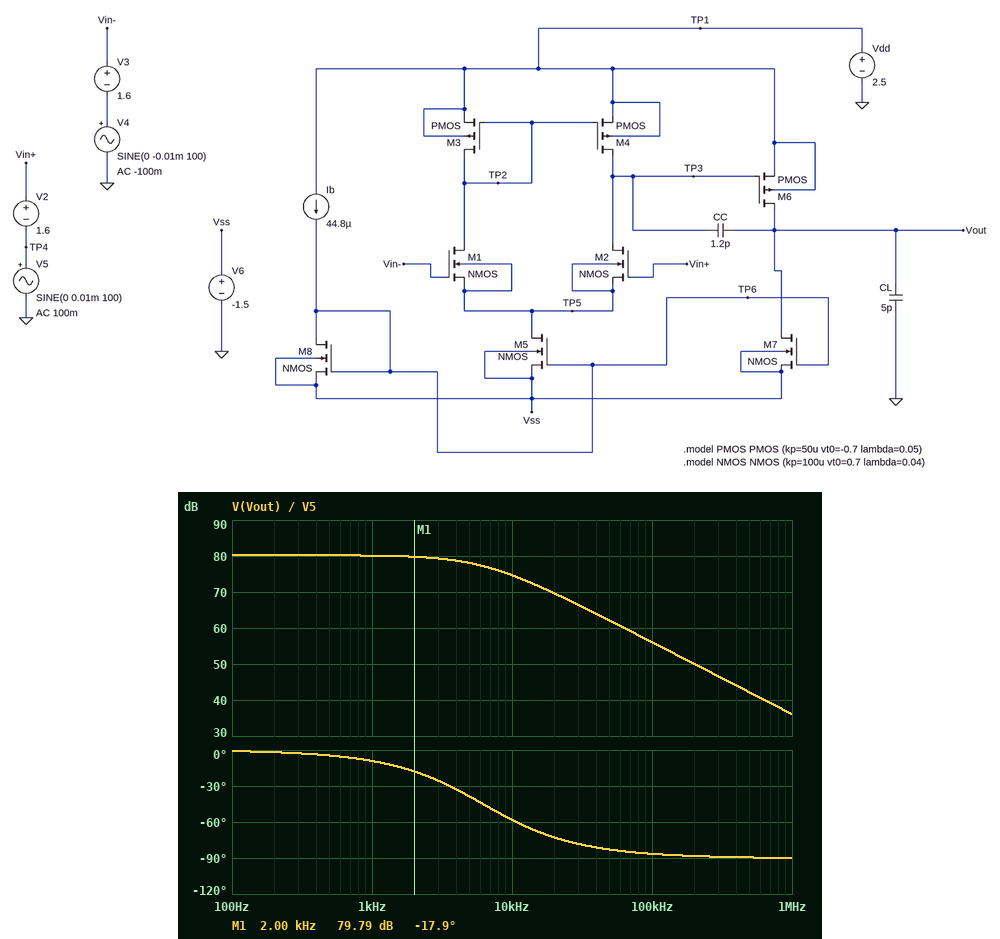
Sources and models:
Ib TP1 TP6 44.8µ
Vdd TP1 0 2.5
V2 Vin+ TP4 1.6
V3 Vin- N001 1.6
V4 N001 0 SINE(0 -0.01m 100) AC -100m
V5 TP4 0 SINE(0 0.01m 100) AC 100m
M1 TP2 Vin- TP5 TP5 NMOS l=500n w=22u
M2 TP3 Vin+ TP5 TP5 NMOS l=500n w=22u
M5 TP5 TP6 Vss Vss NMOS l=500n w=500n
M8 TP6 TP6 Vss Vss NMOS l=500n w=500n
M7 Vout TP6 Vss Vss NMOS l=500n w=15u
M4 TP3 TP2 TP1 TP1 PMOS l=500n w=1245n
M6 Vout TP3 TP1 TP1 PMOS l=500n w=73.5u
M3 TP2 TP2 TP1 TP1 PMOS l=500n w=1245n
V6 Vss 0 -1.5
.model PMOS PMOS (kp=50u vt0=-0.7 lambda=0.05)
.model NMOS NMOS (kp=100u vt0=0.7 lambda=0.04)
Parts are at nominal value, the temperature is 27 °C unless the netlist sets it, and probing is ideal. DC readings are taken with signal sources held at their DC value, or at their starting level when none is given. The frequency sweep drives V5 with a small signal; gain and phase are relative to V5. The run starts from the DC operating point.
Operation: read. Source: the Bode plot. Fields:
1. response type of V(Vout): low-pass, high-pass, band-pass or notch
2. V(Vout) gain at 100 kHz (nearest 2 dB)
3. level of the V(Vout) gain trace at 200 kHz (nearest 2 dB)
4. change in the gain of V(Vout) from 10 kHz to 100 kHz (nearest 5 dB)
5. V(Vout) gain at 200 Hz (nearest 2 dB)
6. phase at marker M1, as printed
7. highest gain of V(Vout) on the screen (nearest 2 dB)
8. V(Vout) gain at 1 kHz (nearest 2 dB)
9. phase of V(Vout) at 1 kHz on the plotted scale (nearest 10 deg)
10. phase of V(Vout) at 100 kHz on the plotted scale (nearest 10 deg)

low-pass
56 dB
50 dB
-20 dB
80 dB
-17.9 deg
80 dB
80 dB
-10 deg
-90 deg
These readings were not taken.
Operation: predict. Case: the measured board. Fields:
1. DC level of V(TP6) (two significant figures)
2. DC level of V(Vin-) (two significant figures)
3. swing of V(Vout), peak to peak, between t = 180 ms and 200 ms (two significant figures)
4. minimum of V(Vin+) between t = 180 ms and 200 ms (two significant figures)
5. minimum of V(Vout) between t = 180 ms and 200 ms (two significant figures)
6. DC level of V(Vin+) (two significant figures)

120 mV
1.6 V
370 mV
1.6 V
650 mV
1.6 V
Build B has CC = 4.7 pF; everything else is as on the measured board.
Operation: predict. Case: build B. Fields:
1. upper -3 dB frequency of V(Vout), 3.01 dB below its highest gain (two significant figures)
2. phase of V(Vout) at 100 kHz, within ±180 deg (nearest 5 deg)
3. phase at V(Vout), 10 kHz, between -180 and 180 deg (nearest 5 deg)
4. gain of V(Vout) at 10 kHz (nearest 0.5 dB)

1.6 kHz
-90 deg
-80 deg
64.0 dB
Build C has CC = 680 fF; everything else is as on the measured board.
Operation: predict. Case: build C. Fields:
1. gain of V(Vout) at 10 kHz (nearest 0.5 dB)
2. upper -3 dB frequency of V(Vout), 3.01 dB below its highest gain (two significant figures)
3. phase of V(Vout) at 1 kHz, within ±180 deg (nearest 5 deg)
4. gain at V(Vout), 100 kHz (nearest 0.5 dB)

77.5 dB
11 kHz
-5 deg
61.0 dB
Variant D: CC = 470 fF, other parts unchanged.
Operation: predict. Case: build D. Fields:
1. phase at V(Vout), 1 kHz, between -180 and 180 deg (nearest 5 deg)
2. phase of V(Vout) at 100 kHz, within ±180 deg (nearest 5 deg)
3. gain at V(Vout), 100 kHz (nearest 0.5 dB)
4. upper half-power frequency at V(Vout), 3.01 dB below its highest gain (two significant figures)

-5 deg
-80 deg
64.0 dB
16 kHz
